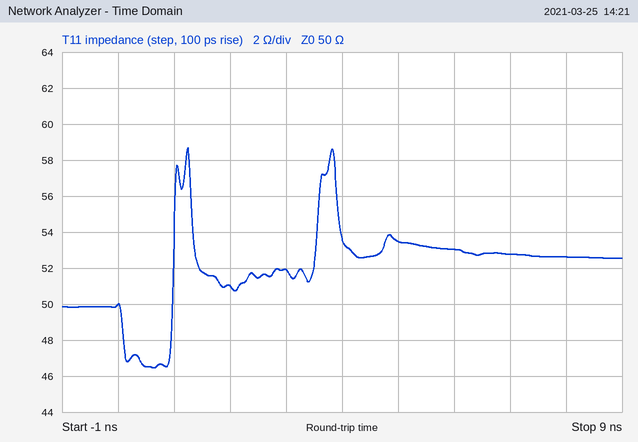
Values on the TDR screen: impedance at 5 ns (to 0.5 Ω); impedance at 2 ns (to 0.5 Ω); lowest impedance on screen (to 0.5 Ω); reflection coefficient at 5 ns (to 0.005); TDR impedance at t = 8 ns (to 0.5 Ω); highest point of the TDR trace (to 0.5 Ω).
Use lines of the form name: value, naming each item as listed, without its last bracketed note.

impedance at 5 ns: 53.5 Ω
impedance at 2 ns: 51.0 Ω
lowest impedance on screen: 46.5 Ω
reflection coefficient at 5 ns: +0.035
TDR impedance at t = 8 ns: 52.5 Ω
highest point of the TDR trace: 58.5 Ω
